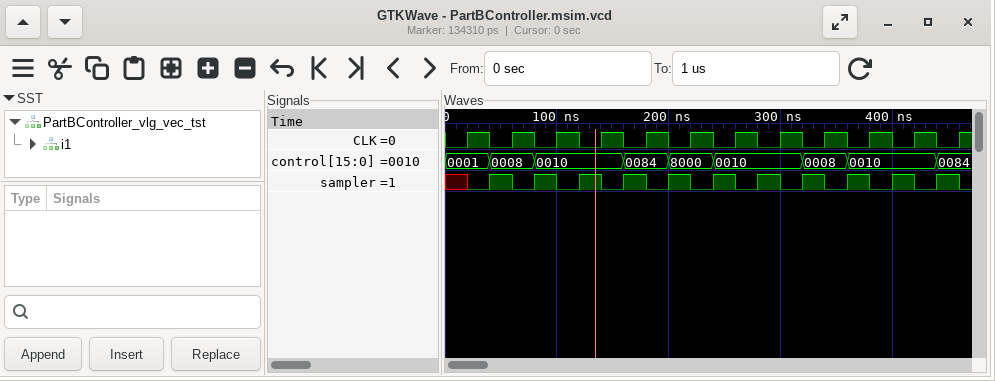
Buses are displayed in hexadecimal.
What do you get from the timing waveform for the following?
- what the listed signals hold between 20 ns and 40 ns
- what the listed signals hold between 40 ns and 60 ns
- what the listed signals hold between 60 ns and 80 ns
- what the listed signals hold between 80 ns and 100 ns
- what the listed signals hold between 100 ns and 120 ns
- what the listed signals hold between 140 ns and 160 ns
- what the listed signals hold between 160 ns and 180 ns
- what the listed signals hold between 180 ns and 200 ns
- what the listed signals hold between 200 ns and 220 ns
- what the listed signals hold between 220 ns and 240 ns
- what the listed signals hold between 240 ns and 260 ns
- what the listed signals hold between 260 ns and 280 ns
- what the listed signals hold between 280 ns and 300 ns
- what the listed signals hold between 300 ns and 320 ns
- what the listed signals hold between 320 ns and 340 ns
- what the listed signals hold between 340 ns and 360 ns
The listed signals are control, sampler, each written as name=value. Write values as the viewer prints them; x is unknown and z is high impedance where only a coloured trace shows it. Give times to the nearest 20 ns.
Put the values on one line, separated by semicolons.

control=0001, sampler=0; control=0008, sampler=1; control=0008, sampler=0; control=0010, sampler=1; control=0010, sampler=0; control=0010, sampler=0; control=0084, sampler=1; control=0084, sampler=0; control=8000, sampler=1; control=8000, sampler=0; control=0010, sampler=1; control=0010, sampler=0; control=0010, sampler=1; control=0010, sampler=0; control=0008, sampler=1; control=0008, sampler=0
